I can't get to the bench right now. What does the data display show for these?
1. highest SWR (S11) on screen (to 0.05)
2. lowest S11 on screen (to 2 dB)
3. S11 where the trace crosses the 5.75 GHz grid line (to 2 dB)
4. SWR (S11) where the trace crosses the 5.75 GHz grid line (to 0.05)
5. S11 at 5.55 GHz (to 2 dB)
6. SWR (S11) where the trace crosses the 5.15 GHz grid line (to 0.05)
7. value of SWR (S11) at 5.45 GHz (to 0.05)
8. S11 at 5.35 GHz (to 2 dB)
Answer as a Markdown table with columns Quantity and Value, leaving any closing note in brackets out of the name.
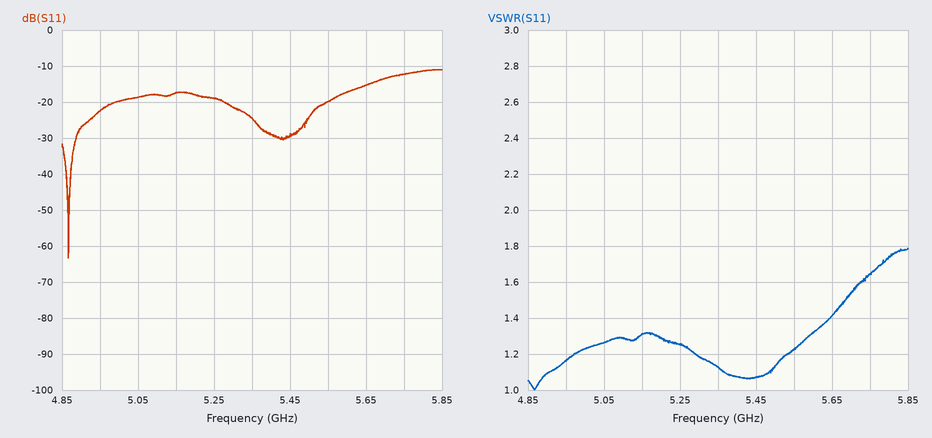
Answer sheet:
| Quantity | Value |
|---|---|
| highest SWR (S11) on screen | 1.80 |
| lowest S11 on screen | -64 dB |
| S11 where the trace crosses the 5.75 GHz grid line | -12 dB |
| SWR (S11) where the trace crosses the 5.75 GHz grid line | 1.65 |
| S11 at 5.55 GHz | -20 dB |
| SWR (S11) where the trace crosses the 5.15 GHz grid line | 1.30 |
| value of SWR (S11) at 5.45 GHz | 1.05 |
| S11 at 5.35 GHz | -24 dB |
